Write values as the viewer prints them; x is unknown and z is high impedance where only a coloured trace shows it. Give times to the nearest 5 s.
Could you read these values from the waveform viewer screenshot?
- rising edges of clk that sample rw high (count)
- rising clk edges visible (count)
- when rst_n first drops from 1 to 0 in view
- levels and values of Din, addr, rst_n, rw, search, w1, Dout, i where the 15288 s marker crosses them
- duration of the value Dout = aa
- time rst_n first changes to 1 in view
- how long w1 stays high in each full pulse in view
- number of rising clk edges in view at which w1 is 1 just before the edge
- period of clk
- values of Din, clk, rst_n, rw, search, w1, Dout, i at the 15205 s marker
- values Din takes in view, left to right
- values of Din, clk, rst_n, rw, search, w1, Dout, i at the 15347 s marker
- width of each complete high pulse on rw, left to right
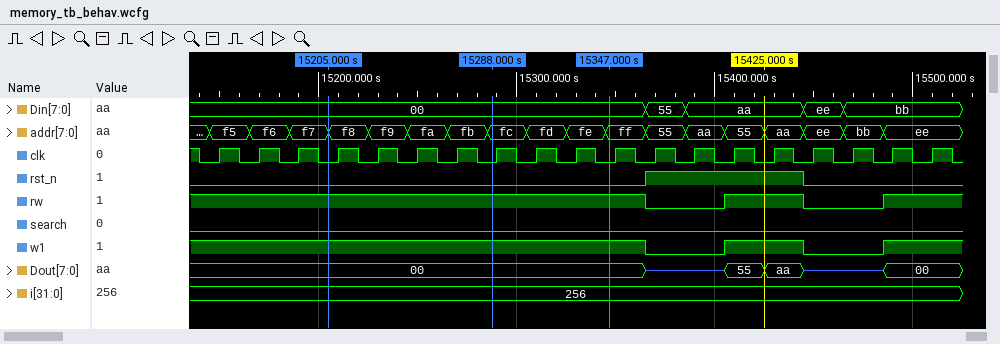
15
19
15445 s
Din=00, addr=fc, rst_n=0, rw=1, search=0, w1=1, Dout=00, i=256
20 s
15365 s
40 s
15
20 s
Din=00, clk=0, rst_n=0, rw=1, search=0, w1=1, Dout=00, i=256
00, 55, aa, ee, bb
Din=00, clk=0, rst_n=0, rw=1, search=0, w1=1, Dout=00, i=256
40 s
